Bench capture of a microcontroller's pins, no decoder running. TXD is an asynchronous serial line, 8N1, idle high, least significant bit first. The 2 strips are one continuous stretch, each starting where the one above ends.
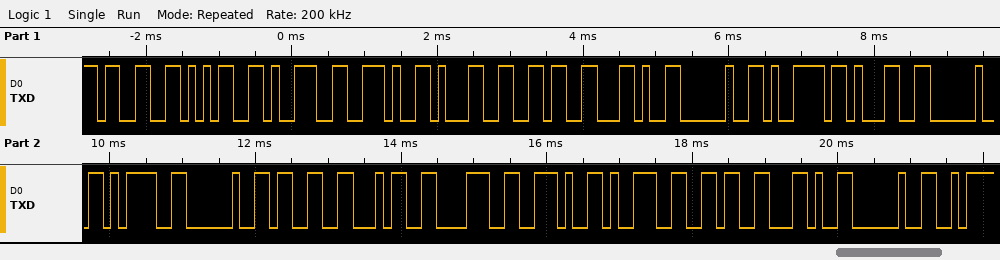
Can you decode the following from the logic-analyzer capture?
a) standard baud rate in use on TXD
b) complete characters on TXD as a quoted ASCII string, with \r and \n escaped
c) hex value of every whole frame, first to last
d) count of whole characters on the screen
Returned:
9600 baud
"359.16, y1 = 348.96, "
33 35 39 2E 31 36 2C 20 79 31 20 3D 20 33 34 38 2E 39 36 2C 20
21
